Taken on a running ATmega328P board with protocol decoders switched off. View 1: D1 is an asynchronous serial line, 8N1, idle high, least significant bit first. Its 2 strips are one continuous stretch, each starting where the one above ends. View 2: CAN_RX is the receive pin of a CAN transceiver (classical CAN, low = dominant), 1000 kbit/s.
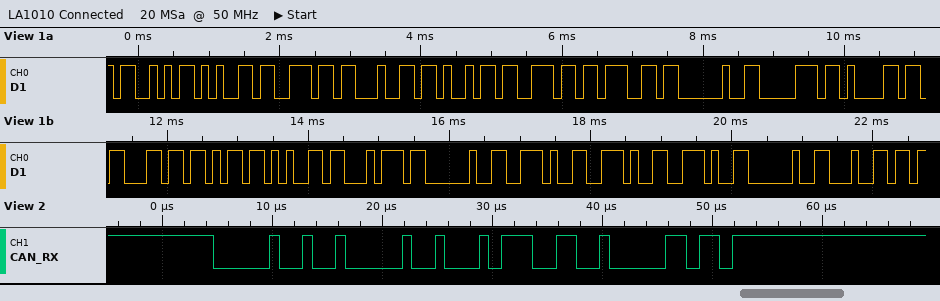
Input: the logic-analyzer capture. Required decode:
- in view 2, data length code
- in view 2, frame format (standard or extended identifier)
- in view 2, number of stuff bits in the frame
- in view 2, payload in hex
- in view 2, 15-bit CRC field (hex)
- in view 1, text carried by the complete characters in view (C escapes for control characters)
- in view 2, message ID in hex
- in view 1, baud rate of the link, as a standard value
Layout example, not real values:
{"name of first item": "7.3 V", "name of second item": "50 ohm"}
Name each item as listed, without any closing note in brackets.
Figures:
{"in view 2, data length code": "1", "in view 2, frame format": "standard", "in view 2, number of stuff bits in the frame": "3", "in view 2, payload in hex": "17", "in view 2, 15-bit CRC field": "0x1905", "in view 1, text carried by the complete characters in view": "\"Sending packet ... d\"", "in view 2, message ID in hex": "0x012", "in view 1, baud rate of the link, as a standard value": "9600 baud"}
